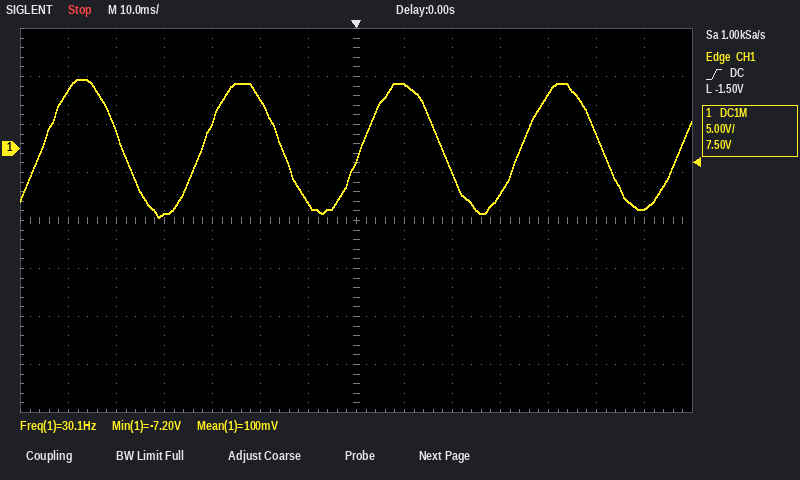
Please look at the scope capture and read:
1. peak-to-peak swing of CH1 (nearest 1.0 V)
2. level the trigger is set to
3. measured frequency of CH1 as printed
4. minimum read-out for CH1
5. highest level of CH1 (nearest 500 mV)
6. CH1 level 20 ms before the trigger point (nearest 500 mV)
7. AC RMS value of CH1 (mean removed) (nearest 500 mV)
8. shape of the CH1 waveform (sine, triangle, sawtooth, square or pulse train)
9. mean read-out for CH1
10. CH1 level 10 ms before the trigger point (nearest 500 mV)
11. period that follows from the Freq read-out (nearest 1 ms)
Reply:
14.0 V
-1.50 V
30.1 Hz
-7.20 V
7.0 V
5.0 V
5.0 V
sine
100 mV
-5.5 V
33 ms
